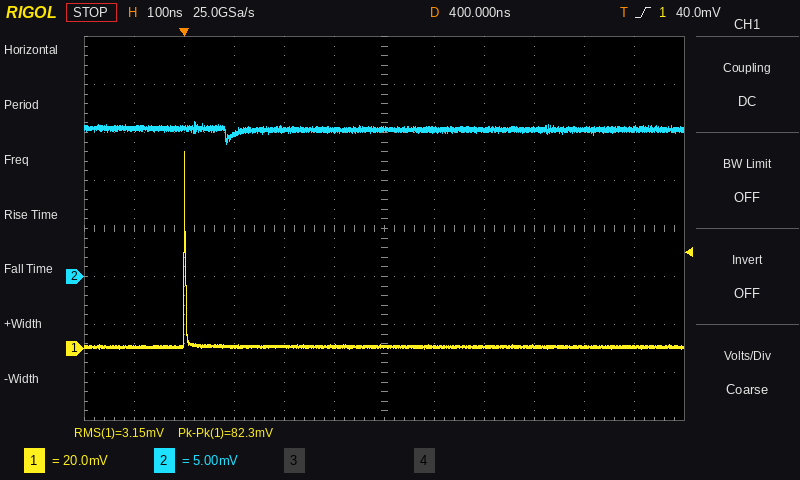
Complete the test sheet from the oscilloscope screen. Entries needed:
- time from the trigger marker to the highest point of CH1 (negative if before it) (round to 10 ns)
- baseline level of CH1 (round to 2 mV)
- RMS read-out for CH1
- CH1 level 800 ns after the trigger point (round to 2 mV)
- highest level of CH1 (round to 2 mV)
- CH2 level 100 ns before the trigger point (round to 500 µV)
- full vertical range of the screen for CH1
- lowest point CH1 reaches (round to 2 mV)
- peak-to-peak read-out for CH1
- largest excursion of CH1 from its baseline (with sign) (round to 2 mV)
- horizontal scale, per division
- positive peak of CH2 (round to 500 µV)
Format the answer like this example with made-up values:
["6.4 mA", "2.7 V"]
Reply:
["0 ns", "0 mV", "3.15 mV", "0 mV", "82 mV", "15.5 mV", "160 mV", "0 mV", "82.3 mV", "+82 mV", "100 ns", "16.0 mV"]
